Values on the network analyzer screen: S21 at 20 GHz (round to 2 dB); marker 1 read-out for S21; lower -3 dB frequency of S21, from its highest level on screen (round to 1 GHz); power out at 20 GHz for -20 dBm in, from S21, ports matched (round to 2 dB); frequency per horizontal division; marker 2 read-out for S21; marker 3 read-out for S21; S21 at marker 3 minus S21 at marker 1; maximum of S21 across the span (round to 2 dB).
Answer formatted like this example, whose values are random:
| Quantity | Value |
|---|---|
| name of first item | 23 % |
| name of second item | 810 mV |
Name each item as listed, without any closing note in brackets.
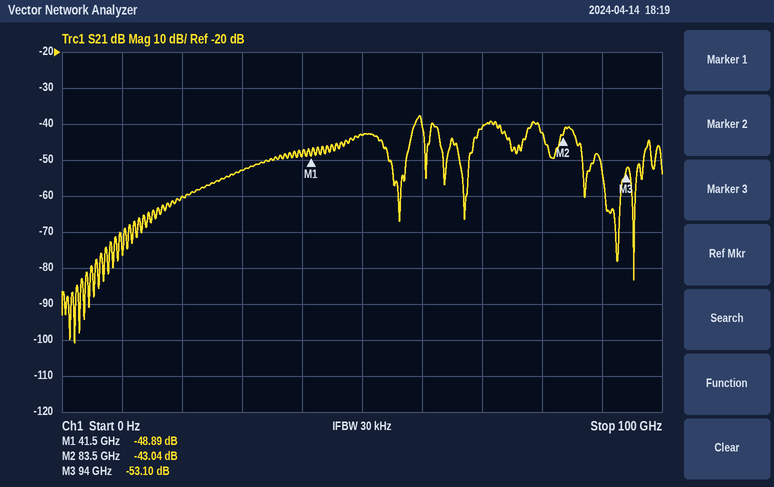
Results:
| Quantity | Value |
|---|---|
| S21 at 20 GHz | -60 dB |
| marker 1 read-out for S21 | -48.89 dB |
| lower -3 dB frequency of S21, from its highest level on screen | 59 GHz |
| power out at 20 GHz for -20 dBm in, from S21, ports matched | -80 dBm |
| frequency per horizontal division | 10 GHz |
| marker 2 read-out for S21 | -43.04 dB |
| marker 3 read-out for S21 | -53.10 dB |
| S21 at marker 3 minus S21 at marker 1 | -4.21 dB |
| maximum of S21 across the span | -38 dB |
